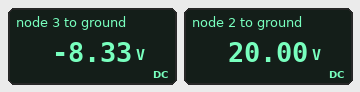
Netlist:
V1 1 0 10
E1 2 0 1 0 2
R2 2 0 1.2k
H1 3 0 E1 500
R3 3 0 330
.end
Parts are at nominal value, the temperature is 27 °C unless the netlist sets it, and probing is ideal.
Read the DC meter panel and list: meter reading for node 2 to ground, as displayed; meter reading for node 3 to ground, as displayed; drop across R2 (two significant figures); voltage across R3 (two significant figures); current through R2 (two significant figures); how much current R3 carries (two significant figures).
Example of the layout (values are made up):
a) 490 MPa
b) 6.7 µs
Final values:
a) 20.00 V
b) -8.33 V
c) 20 V
d) 8.3 V
e) 17 mA
f) 25 mA
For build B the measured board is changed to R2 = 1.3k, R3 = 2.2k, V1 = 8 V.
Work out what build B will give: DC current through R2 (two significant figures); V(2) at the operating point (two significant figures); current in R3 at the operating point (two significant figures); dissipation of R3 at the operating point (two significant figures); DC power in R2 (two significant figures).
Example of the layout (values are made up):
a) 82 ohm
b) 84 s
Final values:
a) 12 mA
b) 16 V
c) 2.8 mA
d) 17 mW
e) 200 mW
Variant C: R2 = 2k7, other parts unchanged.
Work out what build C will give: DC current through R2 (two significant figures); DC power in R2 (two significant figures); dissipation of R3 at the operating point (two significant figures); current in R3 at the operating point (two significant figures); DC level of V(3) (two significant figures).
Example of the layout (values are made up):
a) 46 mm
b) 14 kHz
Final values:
a) 7.4 mA
b) 150 mW
c) 42 mW
d) 11 mA
e) -3.7 V
